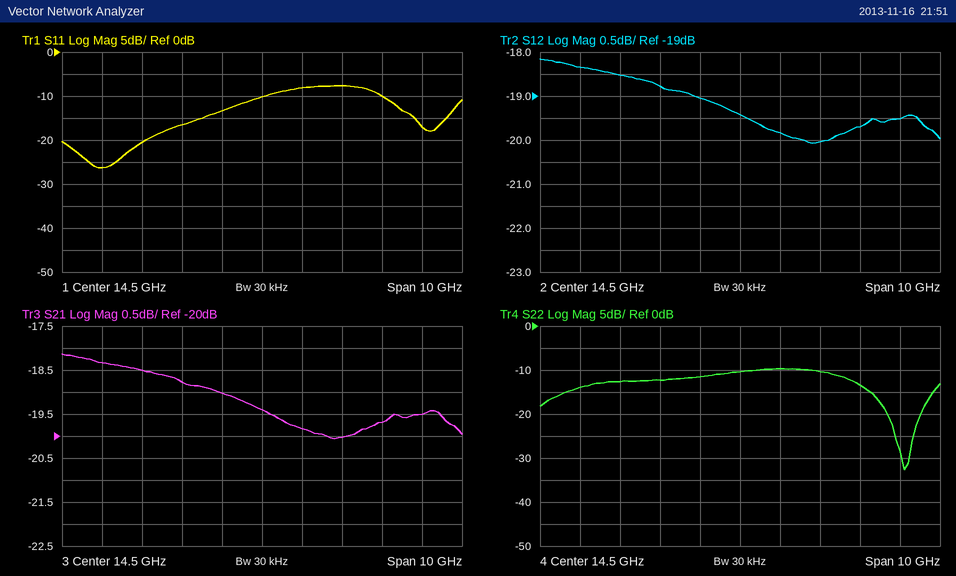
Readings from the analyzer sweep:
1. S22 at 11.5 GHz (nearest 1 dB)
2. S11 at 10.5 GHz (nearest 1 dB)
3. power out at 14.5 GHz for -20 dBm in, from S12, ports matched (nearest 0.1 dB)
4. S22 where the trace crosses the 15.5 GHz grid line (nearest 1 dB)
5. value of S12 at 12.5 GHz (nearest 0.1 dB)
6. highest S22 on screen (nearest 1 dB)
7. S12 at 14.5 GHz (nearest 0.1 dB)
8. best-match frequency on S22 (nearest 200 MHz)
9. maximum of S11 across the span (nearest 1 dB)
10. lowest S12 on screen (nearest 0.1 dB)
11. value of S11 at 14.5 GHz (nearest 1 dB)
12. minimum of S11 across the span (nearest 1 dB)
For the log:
-13 dB
-26 dB
-39.4 dBm
-10 dB
-18.8 dB
-10 dB
-19.4 dB
18.6 GHz
-8 dB
-20.1 dB
-10 dB
-26 dB
